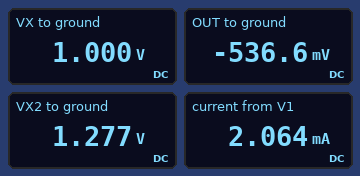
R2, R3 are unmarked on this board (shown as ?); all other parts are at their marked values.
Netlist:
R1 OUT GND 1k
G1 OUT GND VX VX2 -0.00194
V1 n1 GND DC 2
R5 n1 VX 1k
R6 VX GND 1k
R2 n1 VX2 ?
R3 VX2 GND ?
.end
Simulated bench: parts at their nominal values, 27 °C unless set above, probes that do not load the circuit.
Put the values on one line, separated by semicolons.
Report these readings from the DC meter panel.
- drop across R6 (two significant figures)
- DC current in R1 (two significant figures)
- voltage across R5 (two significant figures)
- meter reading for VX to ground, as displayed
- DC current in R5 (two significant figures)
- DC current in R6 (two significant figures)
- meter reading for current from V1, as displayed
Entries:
1.0 V; 540 µA; 1.0 V; 1.000 V; 1.0 mA; 1.0 mA; 2.064 mA
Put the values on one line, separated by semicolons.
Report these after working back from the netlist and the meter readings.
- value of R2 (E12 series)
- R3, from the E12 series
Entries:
680 Ω; 1.2 kΩ
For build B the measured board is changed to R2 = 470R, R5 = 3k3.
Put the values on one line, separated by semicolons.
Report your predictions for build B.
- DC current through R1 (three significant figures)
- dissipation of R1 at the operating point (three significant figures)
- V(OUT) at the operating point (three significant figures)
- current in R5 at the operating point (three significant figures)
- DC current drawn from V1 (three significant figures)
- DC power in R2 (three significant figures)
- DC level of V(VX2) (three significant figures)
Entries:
1.89 mA; 3.56 mW; -1.89 V; 465 µA; 1.66 mA; 674 µW; 1.44 V
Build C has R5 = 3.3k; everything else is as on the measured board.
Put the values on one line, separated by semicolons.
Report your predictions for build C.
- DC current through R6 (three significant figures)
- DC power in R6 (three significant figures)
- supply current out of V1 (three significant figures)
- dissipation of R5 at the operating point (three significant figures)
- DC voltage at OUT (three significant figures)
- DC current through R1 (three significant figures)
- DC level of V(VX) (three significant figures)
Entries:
465 µA; 216 µW; 1.53 mA; 714 µW; -1.57 V; 1.57 mA; 465 mV
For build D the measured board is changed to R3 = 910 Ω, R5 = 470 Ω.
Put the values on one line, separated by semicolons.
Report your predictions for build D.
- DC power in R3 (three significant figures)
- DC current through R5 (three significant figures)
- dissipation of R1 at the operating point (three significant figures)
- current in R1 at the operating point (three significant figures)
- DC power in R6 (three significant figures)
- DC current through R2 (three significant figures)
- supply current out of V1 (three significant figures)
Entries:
1.44 mW; 1.36 mA; 175 µW; 419 µA; 1.85 mW; 1.26 mA; 2.62 mA
